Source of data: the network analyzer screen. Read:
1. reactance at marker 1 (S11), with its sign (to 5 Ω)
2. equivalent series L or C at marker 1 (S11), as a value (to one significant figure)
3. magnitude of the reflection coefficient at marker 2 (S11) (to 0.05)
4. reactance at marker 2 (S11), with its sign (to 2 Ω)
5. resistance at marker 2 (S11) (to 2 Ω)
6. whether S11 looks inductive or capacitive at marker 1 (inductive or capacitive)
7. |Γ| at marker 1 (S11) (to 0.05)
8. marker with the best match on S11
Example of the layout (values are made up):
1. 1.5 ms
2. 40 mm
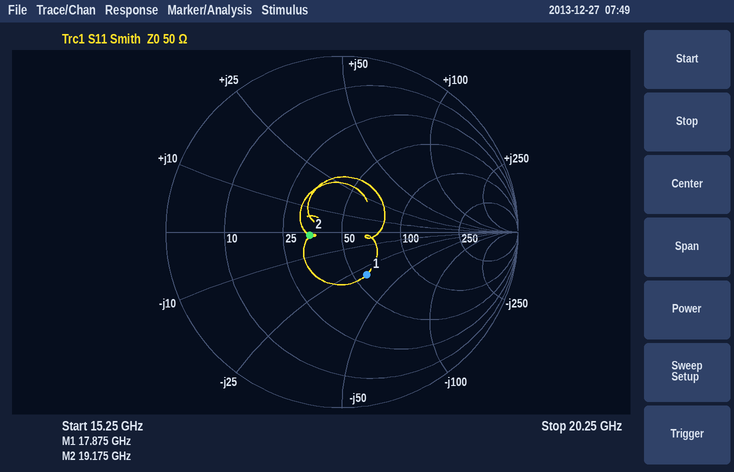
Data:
1. -30 Ω
2. 300 fF
3. 0.20
4. -2 Ω
5. 34 Ω
6. capacitive
7. 0.30
8. marker 2
